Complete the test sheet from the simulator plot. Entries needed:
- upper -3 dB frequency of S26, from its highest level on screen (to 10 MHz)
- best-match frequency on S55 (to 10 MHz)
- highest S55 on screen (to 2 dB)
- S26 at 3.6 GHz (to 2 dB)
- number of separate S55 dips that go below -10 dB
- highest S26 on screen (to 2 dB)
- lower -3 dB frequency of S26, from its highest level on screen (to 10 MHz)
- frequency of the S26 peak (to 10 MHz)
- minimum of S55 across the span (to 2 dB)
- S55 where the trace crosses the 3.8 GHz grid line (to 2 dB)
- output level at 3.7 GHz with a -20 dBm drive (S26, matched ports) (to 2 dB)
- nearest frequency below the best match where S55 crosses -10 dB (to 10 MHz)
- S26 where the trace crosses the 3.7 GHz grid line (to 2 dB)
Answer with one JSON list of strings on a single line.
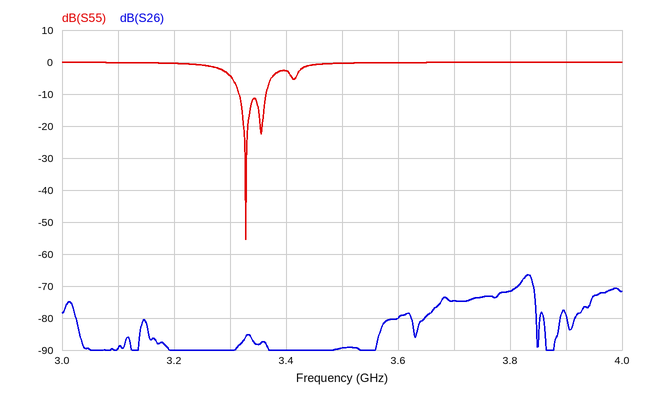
["3.84 GHz", "3.33 GHz", "0 dB", "-80 dB", "2", "-66 dB", "3.82 GHz", "3.83 GHz", "-56 dB", "0 dB", "-94 dBm", "3.32 GHz", "-74 dB"]
